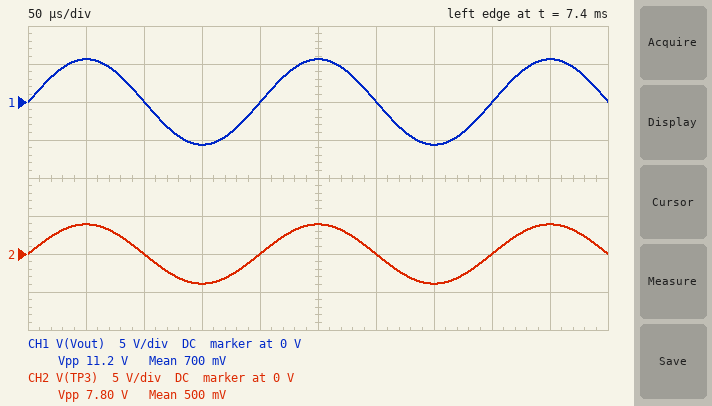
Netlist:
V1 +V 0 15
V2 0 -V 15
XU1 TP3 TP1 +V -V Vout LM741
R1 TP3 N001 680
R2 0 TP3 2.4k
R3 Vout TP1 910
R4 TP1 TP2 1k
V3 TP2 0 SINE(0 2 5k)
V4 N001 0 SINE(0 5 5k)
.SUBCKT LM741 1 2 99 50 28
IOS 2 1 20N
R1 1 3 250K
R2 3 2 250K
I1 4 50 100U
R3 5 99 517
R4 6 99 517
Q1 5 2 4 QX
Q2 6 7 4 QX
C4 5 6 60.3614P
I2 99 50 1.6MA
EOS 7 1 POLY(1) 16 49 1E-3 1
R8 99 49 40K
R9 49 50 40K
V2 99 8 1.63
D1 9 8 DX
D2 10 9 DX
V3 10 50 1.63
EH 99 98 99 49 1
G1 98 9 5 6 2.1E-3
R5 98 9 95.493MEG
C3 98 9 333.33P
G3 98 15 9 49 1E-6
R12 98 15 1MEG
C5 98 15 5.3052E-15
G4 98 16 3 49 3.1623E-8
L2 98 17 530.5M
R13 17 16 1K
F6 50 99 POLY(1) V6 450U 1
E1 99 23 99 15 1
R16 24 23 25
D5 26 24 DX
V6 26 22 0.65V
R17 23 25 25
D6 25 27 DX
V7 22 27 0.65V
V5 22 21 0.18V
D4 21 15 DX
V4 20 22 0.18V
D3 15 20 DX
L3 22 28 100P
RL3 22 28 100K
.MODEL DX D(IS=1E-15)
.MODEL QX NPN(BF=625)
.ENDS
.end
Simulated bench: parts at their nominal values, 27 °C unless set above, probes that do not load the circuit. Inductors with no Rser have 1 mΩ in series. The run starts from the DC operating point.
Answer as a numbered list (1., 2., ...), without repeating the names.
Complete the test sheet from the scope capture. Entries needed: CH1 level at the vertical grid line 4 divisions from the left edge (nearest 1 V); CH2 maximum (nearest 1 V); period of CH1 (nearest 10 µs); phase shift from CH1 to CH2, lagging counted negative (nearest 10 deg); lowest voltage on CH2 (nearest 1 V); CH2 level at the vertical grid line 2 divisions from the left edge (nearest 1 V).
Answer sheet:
1. 0 V
2. 4 V
3. 200 µs
4. 0 deg
5. -4 V
6. 0 V
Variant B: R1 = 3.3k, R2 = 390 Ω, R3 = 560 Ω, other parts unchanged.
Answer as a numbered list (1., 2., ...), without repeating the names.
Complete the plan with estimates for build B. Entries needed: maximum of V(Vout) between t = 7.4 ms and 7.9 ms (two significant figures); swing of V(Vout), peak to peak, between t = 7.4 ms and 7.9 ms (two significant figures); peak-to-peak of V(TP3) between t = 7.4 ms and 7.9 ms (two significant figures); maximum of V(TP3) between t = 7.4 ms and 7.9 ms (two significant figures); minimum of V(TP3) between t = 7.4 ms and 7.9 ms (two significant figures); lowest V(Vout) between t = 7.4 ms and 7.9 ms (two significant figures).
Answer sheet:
1. 300 mV
2. 590 mV
3. 1.1 V
4. 530 mV
5. -530 mV
6. -290 mV
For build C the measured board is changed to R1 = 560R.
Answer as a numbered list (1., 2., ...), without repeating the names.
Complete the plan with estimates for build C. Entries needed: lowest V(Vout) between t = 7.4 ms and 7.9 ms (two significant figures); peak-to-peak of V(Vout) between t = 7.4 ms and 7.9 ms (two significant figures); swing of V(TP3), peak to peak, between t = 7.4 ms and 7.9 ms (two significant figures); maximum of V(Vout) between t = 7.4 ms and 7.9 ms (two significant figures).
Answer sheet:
1. -5.9 V
2. 12 V
3. 8.1 V
4. 5.9 V
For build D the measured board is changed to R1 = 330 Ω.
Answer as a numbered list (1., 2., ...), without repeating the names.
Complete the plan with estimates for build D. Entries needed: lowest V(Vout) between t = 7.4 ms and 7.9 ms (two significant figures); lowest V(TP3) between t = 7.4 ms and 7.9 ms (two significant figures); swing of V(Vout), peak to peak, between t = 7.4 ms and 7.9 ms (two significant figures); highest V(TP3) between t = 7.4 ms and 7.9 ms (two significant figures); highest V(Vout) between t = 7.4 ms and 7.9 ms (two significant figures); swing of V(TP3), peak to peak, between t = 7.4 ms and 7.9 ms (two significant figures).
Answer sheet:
1. -6.6 V
2. -4.4 V
3. 13 V
4. 4.4 V
5. 6.6 V
6. 8.8 V
